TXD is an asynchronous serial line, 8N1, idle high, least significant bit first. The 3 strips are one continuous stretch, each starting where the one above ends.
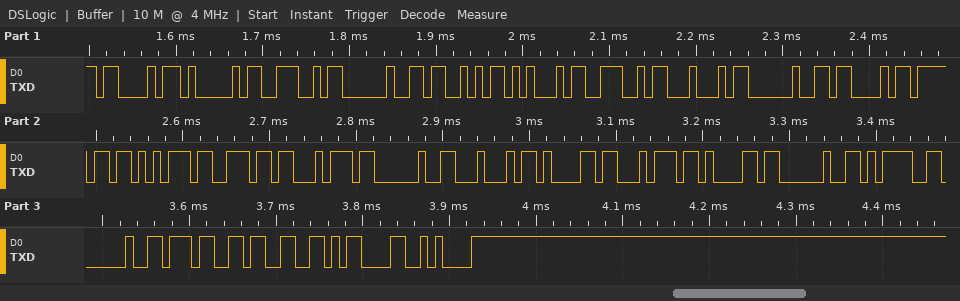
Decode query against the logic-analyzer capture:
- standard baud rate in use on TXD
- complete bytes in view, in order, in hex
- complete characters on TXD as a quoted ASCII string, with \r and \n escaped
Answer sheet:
115200 baud
43 41 4E 20 53 45 4E 44 20 43 6F 75 6E 74 20 44 61 74 61 20 3D 20 37 33 0D 0A
"CAN SEND Count Data = 73\r\n"
